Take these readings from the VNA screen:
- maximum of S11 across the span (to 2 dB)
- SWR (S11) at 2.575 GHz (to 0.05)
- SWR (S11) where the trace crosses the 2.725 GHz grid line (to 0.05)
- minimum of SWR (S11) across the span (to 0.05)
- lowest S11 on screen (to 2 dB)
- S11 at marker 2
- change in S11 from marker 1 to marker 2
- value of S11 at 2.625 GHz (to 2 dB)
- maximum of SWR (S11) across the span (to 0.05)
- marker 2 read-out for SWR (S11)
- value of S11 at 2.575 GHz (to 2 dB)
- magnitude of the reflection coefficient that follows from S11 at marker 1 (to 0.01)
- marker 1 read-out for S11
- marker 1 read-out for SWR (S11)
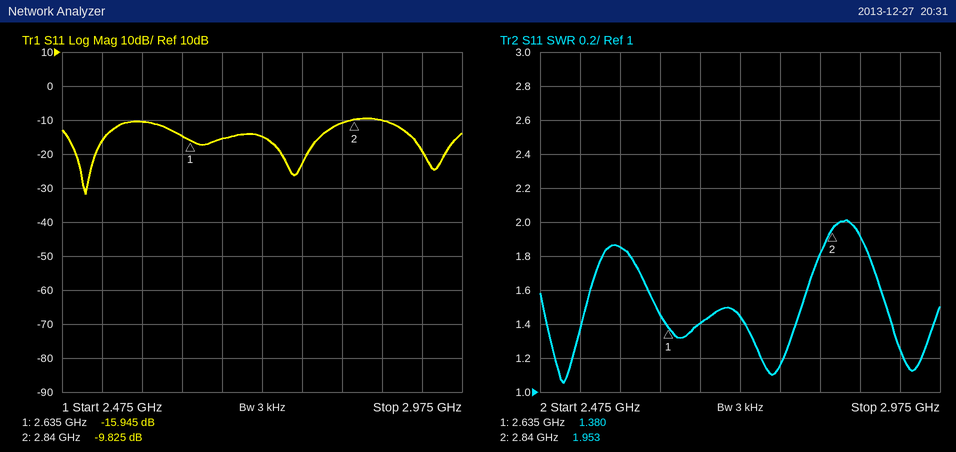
-10 dB
1.85
1.45
1.05
-32 dB
-9.825 dB
6.120 dB
-14 dB
2.00
1.953
-10 dB
0.16
-15.945 dB
1.380
